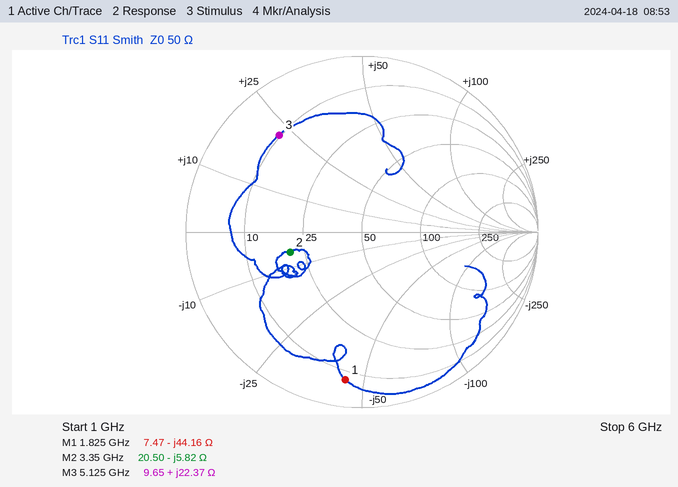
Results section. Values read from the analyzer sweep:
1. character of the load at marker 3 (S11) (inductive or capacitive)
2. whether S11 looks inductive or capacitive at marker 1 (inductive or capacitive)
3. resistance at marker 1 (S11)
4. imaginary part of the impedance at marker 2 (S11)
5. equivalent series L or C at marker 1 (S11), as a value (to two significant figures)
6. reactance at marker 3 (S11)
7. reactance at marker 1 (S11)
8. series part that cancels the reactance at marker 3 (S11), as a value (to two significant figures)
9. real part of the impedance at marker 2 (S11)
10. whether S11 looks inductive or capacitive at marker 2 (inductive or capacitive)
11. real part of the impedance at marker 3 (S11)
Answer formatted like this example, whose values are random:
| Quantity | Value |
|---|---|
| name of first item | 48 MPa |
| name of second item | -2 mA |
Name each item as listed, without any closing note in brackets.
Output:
| Quantity | Value |
|---|---|
| character of the load at marker 3 (S11) | inductive |
| whether S11 looks inductive or capacitive at marker 1 | capacitive |
| resistance at marker 1 | 7.47 Ω |
| imaginary part of the impedance at marker 2 | -5.82 Ω |
| equivalent series L or C at marker 1 (S11), as a value | 2.0 pF |
| reactance at marker 3 | +22.37 Ω |
| reactance at marker 1 | -44.16 Ω |
| series part that cancels the reactance at marker 3 (S11), as a value | 1.4 pF |
| real part of the impedance at marker 2 | 20.50 Ω |
| whether S11 looks inductive or capacitive at marker 2 | capacitive |
| real part of the impedance at marker 3 | 9.65 Ω |
